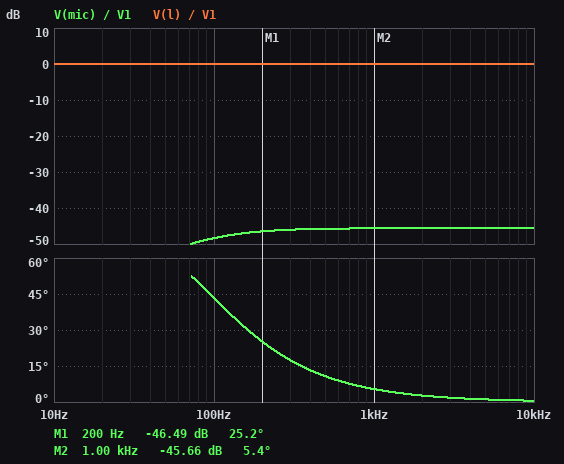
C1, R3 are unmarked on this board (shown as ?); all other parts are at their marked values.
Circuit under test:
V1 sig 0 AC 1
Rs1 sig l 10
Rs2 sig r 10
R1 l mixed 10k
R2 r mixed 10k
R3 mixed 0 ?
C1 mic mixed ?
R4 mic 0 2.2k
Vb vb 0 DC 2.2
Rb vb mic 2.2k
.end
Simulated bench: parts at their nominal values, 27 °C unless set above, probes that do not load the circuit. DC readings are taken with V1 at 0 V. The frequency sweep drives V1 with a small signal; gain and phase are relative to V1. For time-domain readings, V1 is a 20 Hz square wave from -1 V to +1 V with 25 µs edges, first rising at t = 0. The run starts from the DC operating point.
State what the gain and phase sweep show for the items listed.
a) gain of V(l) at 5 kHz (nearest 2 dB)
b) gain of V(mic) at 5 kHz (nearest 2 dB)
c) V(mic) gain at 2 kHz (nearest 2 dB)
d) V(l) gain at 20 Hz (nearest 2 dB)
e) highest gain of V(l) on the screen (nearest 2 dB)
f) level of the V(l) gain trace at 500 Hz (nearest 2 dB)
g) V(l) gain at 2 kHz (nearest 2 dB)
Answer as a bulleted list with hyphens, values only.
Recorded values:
- 0 dB
- -46 dB
- -46 dB
- 0 dB
- 0 dB
- 0 dB
- 0 dB
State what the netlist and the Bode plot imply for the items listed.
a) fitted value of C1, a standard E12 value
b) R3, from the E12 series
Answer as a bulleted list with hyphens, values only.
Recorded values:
- 1.5 µF
- 27 Ω
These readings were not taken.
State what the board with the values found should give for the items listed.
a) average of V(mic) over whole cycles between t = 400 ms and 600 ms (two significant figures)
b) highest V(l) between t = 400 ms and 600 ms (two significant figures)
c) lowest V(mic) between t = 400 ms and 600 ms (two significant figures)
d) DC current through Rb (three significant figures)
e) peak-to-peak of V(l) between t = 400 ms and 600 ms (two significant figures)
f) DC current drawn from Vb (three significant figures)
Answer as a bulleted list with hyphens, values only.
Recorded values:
- 1.1 V
- 1.0 V
- 1.1 V
- 500 µA
- 2.0 V
- 500 µA
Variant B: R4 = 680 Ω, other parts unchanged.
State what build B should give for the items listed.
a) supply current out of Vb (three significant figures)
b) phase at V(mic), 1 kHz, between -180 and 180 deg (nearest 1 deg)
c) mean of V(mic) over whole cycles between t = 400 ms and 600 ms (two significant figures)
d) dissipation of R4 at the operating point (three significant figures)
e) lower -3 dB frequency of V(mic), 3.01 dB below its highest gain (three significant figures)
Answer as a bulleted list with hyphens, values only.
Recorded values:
- 764 µA
- 11 deg
- 520 mV
- 397 µW
- 194 Hz
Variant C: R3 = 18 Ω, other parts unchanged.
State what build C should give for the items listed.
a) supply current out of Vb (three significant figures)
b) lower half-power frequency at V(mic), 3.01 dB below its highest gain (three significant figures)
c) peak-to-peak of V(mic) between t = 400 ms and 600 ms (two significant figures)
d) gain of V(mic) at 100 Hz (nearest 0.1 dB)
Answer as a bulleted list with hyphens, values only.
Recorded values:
- 500 µA
- 94.9 Hz
- 14 mV
- -51.8 dB
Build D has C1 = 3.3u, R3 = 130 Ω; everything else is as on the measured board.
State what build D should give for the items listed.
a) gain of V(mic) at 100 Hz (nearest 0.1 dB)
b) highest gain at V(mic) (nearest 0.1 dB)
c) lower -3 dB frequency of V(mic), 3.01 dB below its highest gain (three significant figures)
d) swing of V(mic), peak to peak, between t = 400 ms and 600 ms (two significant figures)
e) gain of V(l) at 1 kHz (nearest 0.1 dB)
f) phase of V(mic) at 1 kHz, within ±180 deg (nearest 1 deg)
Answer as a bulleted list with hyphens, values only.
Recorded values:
- -33.5 dB
- -32.9 dB
- 39.3 Hz
- 90 mV
- 0 dB
- 2 deg
